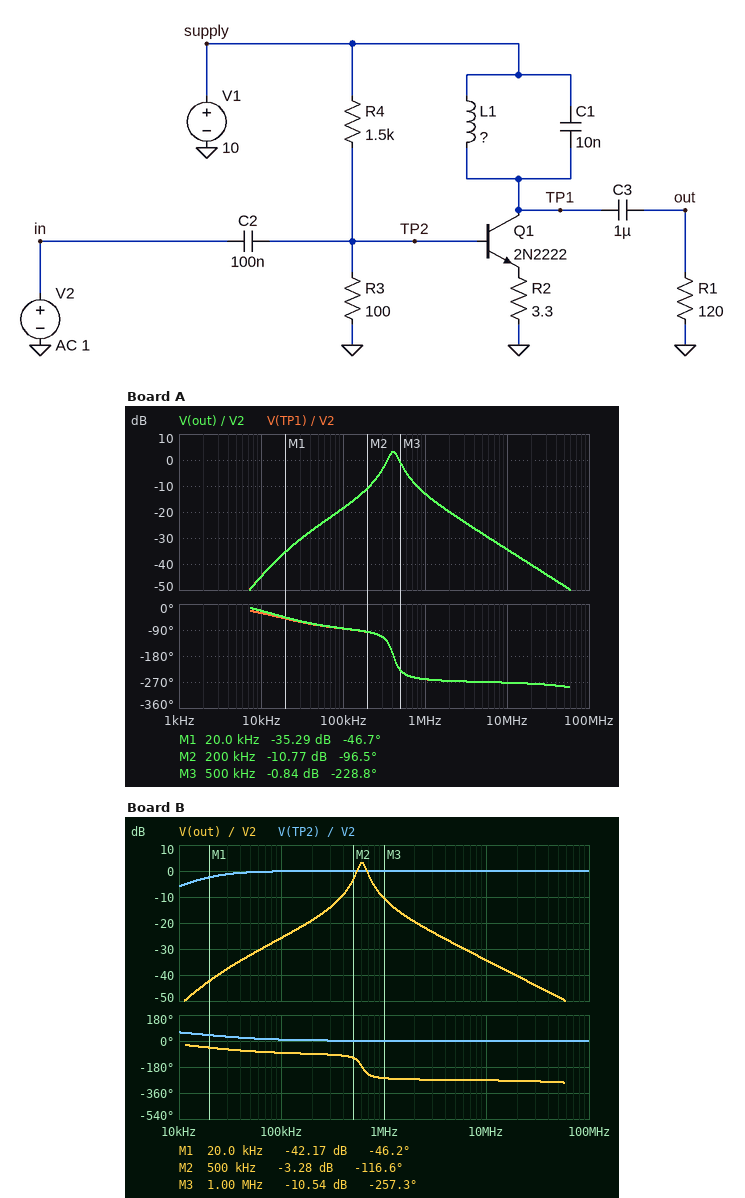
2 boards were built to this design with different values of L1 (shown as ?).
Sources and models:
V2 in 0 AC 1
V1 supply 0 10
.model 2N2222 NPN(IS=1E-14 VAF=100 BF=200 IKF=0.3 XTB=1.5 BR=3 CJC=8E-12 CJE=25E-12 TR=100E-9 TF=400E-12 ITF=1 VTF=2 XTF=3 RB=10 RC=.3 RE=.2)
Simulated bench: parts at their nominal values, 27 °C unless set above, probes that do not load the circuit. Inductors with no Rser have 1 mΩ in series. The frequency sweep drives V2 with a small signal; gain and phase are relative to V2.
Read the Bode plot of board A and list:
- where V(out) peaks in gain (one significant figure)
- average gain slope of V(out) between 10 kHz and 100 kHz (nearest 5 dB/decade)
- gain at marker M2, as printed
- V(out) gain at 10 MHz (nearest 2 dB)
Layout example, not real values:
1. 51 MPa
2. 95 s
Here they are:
1. 400 kHz
2. 25 dB/decade
3. -10.77 dB
4. -34 dB
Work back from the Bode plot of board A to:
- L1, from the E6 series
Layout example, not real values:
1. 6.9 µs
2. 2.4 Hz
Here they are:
1. 15 µH
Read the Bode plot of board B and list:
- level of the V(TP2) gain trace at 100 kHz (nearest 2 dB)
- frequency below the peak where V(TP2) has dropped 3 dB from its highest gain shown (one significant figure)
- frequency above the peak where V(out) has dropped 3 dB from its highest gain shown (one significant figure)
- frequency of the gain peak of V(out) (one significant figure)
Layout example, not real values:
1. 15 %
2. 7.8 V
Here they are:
1. 0 dB
2. 20 kHz
3. 700 kHz
4. 600 kHz
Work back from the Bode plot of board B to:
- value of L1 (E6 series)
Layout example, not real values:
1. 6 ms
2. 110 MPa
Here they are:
1. 6.8 µH
